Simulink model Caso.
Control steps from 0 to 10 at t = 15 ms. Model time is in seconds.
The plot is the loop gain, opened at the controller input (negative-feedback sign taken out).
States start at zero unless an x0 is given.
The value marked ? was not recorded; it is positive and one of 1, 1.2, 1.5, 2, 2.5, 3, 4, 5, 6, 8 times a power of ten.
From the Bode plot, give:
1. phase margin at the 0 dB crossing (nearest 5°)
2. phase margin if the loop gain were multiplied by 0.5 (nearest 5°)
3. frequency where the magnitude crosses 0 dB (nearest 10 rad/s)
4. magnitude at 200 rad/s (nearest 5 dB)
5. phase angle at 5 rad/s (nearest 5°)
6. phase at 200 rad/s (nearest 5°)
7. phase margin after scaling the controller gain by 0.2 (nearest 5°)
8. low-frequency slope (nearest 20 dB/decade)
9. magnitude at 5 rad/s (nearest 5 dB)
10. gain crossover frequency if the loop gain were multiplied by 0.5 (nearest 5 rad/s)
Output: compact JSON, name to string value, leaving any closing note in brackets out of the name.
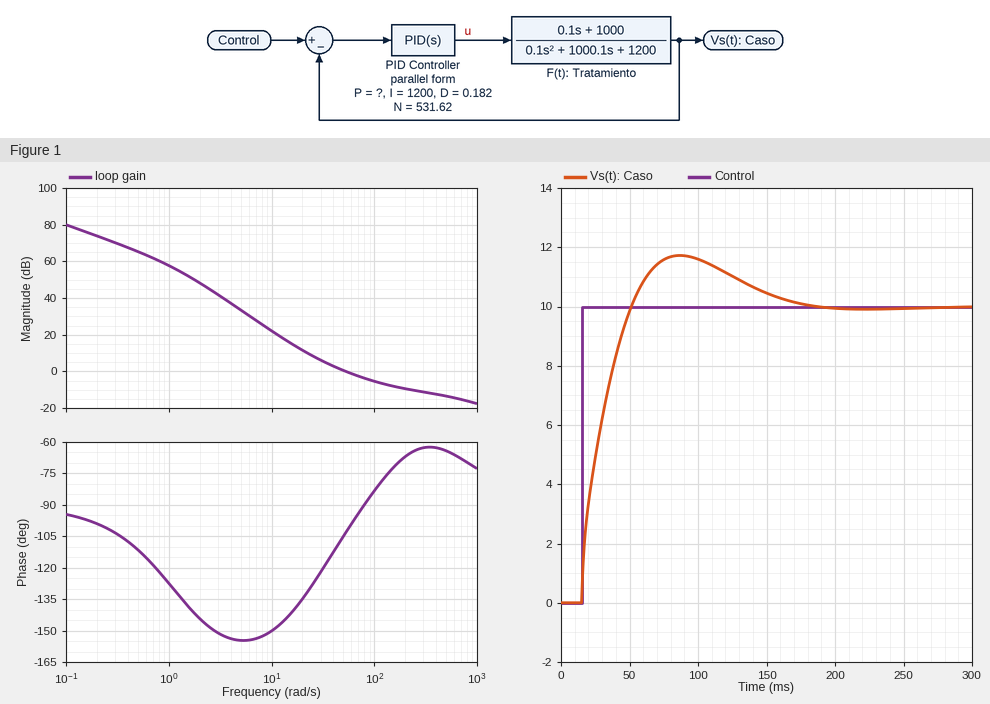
{"phase margin at the 0 dB crossing": "75°", "phase margin if the loop gain were multiplied by 0.5": "60°", "frequency where the magnitude crosses 0 dB": "50 rad/s", "magnitude at 200 rad/s": "-10 dB", "phase angle at 5 rad/s": "-155°", "phase at 200 rad/s": "-65°", "phase margin after scaling the controller gain by 0.2": "40°", "low-frequency slope": "-20 dB/decade", "magnitude at 5 rad/s": "35 dB", "gain crossover frequency if the loop gain were multiplied by 0.5": "30 rad/s"}
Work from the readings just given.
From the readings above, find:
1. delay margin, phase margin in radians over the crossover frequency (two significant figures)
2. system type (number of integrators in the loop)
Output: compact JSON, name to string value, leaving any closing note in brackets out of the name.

{"delay margin, phase margin in radians over the crossover frequency": "0.026 s", "system type": "1"}
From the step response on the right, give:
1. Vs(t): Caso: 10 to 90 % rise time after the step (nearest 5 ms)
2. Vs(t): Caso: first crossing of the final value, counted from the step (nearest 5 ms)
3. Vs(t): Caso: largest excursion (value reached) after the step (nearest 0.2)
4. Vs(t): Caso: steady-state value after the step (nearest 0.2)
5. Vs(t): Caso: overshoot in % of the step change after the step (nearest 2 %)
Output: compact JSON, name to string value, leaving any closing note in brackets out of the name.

{"Vs(t): Caso: 10 to 90 % rise time after the step": "30 ms", "Vs(t): Caso: first crossing of the final value, counted from the step": "35 ms", "Vs(t): Caso: largest excursion (value reached) after the step": "11.8", "Vs(t): Caso: steady-state value after the step": "10.0", "Vs(t): Caso: overshoot in % of the step change after the step": "18 %"}
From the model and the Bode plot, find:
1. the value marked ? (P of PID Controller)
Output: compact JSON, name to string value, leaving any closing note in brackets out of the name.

{"the value marked ?": "50"}
